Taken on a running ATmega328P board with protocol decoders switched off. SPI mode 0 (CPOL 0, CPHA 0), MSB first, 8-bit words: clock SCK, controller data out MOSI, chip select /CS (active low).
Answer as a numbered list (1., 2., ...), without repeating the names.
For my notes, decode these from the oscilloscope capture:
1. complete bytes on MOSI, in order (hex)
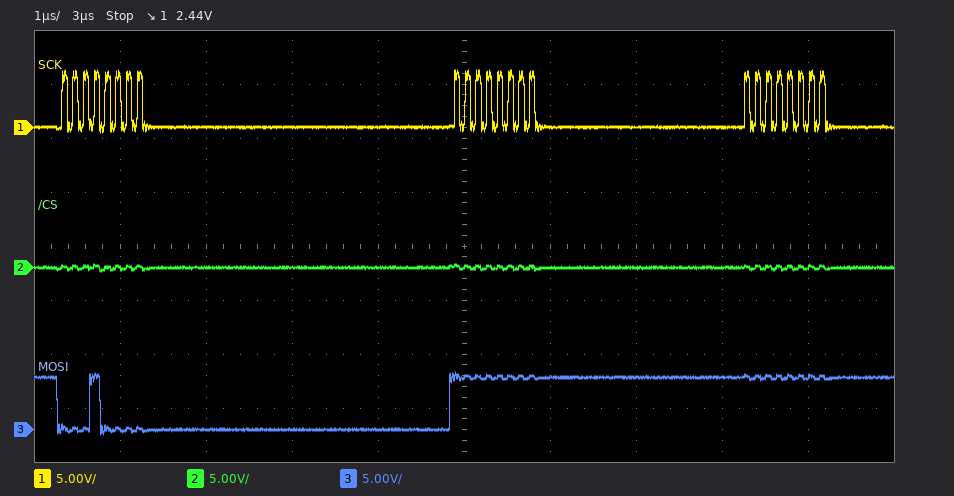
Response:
1. 10 FF FF
